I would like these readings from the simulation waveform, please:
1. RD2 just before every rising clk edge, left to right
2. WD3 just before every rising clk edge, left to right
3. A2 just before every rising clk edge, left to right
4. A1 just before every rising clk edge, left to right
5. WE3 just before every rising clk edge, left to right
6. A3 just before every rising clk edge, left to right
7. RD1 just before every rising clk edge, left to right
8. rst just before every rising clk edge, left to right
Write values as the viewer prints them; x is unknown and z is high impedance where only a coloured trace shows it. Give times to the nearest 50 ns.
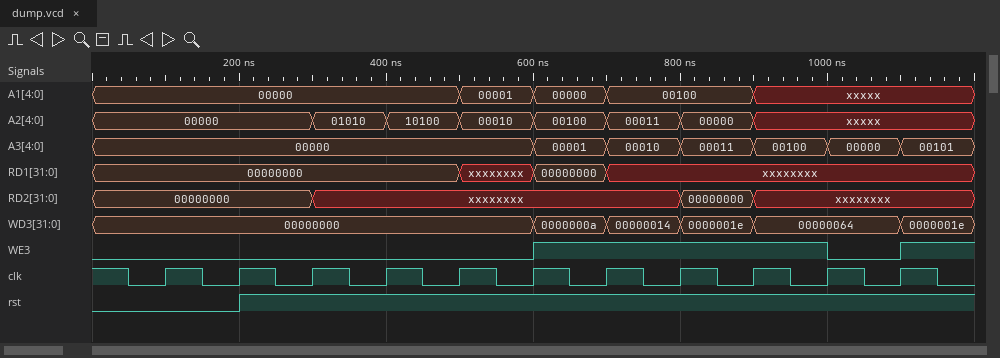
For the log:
00000000, 00000000, 00000000, xxxxxxxx, xxxxxxxx, xxxxxxxx, xxxxxxxx, xxxxxxxx, 00000000, xxxxxxxx, xxxxxxxx
00000000, 00000000, 00000000, 00000000, 00000000, 00000000, 0000000a, 00000014, 0000001e, 00000064, 00000064
00000, 00000, 00000, 01010, 10100, 00010, 00100, 00011, 00000, xxxxx, xxxxx
00000, 00000, 00000, 00000, 00000, 00001, 00000, 00100, 00100, xxxxx, xxxxx
0 0 0 0 0 0 1 1 1 1 0
00000, 00000, 00000, 00000, 00000, 00000, 00001, 00010, 00011, 00100, 00000
00000000, 00000000, 00000000, 00000000, 00000000, xxxxxxxx, 00000000, xxxxxxxx, xxxxxxxx, xxxxxxxx, xxxxxxxx
0 0 1 1 1 1 1 1 1 1 1
